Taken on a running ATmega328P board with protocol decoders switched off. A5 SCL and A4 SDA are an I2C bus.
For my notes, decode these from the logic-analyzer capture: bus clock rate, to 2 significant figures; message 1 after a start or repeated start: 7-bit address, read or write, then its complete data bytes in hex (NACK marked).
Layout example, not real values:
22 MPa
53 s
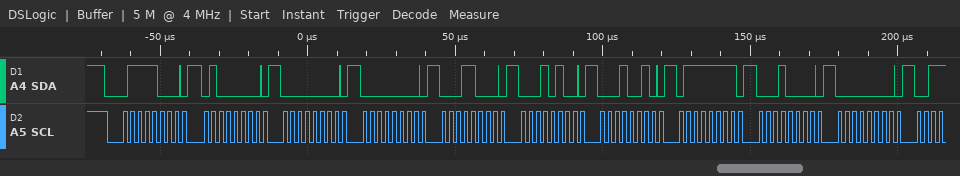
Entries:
400 kHz
0x3C write: 40 00 00 18 14 12 7F 10 00
